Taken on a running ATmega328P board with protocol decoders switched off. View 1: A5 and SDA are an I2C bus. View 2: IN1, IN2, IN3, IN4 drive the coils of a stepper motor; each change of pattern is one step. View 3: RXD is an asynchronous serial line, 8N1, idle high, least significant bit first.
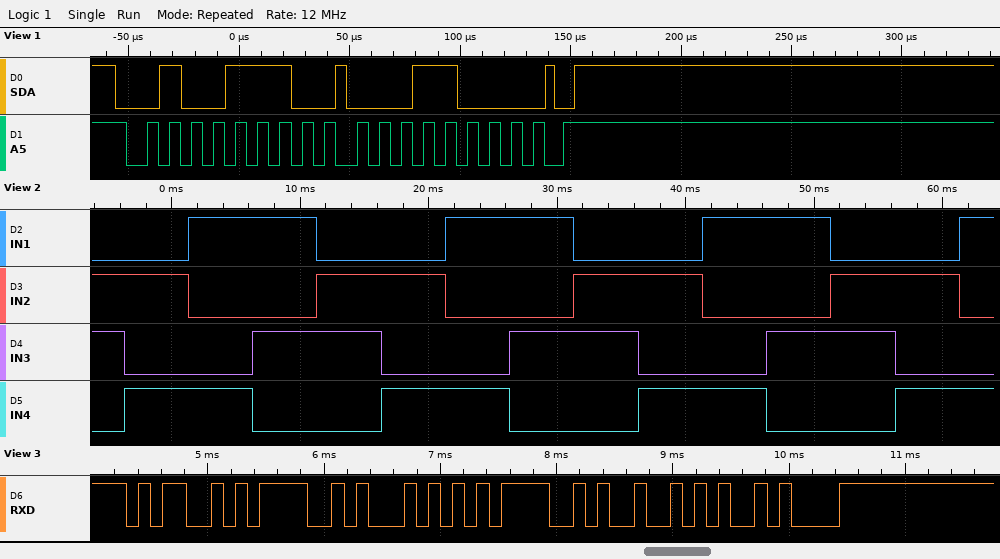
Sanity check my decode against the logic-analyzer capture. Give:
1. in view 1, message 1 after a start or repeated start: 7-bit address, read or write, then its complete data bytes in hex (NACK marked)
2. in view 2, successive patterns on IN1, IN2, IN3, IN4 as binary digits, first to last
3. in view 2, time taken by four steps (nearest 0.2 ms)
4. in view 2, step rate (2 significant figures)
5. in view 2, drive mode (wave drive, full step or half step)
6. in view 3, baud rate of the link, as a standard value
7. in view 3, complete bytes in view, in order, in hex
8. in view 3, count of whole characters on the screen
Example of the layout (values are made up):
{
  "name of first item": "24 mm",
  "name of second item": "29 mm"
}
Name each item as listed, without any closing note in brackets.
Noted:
{
  "in view 1, message 1 after a start or repeated start: 7-bit address, read or write, then its complete data bytes in hex": "0x27 write: 18",
  "in view 2, successive patterns on IN1, IN2, IN3, IN4 as binary digits, first to last": "0110 0101 1001 1010 0110 0101 1001 1010 0110 0101 1001 1010 0110 0101 1001",
  "in view 2, time taken by four steps": "20.0 ms",
  "in view 2, step rate": "200 steps/s",
  "in view 2, drive mode": "full step",
  "in view 3, baud rate of the link, as a standard value": "9600 baud",
  "in view 3, complete bytes in view, in order, in hex": "4D 4F 54 4F 52 0A",
  "in view 3, count of whole characters on the screen": "6"
}
